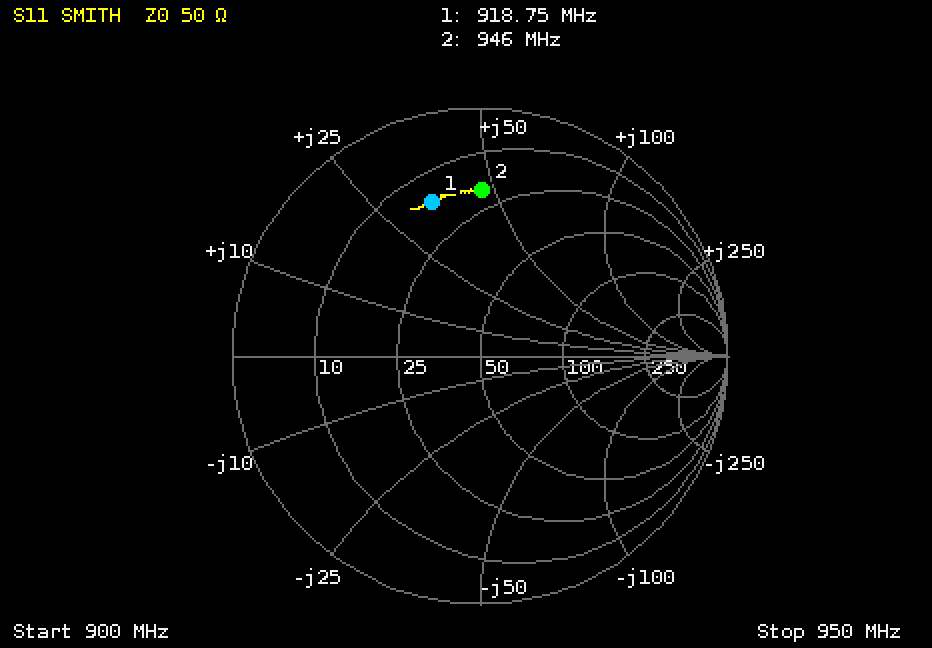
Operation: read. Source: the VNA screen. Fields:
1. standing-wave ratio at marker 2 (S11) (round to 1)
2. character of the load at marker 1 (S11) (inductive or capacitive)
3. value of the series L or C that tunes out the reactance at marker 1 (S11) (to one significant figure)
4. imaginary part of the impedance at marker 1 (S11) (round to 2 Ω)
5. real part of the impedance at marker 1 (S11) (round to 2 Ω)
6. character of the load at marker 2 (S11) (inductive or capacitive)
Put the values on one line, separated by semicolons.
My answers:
5; inductive; 5 pF; +34 Ω; 16 Ω; inductive
